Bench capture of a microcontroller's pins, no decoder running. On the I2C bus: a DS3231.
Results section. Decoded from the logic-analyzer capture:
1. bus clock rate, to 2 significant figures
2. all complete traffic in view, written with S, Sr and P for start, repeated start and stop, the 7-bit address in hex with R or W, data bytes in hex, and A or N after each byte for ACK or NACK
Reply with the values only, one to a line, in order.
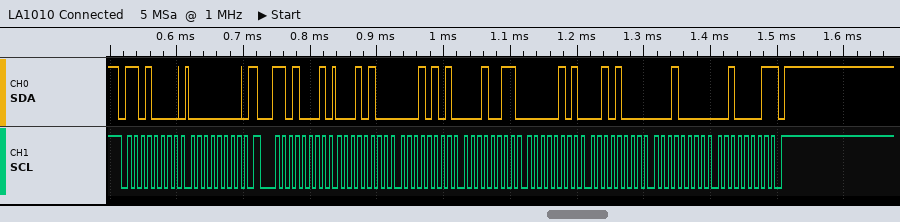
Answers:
100 kHz
S 68W A 00 A Sr 68R A 14 A 15 A 13 A 05 A 28 A 10 A 21 N P
